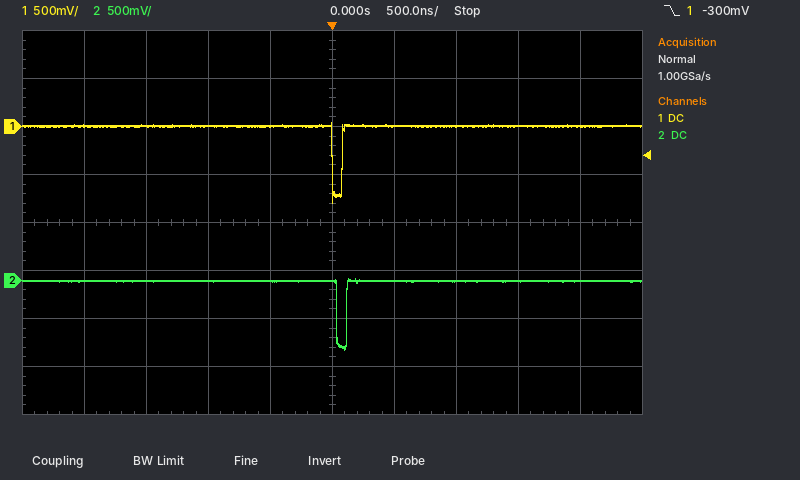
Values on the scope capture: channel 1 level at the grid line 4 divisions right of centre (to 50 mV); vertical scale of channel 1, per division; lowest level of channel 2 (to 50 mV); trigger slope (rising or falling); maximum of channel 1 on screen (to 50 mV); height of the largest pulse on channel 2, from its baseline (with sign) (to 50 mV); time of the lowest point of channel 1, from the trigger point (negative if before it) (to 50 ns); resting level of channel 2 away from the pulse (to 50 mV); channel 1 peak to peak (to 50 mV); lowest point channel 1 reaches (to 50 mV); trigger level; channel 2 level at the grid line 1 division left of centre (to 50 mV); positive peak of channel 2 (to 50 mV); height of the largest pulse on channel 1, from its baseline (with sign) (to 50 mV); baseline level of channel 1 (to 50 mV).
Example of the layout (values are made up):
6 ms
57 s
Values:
0 mV
500 mV
-700 mV
falling
50 mV
-700 mV
0 ns
0 mV
850 mV
-800 mV
-300 mV
0 mV
0 mV
-800 mV
0 mV
